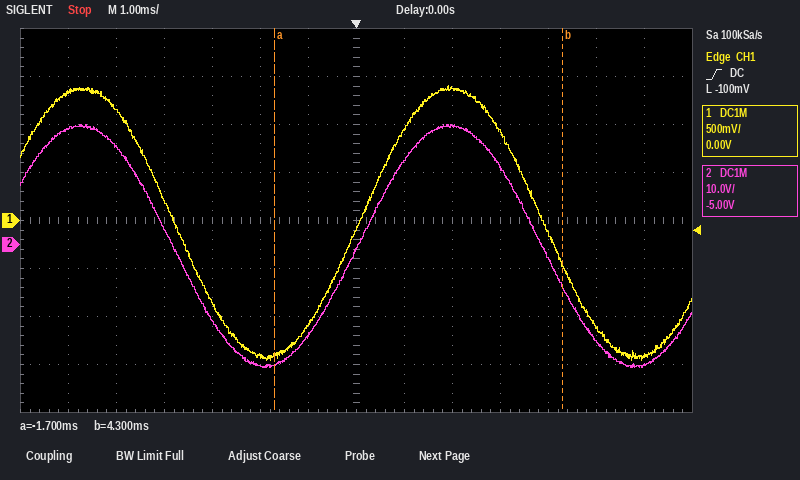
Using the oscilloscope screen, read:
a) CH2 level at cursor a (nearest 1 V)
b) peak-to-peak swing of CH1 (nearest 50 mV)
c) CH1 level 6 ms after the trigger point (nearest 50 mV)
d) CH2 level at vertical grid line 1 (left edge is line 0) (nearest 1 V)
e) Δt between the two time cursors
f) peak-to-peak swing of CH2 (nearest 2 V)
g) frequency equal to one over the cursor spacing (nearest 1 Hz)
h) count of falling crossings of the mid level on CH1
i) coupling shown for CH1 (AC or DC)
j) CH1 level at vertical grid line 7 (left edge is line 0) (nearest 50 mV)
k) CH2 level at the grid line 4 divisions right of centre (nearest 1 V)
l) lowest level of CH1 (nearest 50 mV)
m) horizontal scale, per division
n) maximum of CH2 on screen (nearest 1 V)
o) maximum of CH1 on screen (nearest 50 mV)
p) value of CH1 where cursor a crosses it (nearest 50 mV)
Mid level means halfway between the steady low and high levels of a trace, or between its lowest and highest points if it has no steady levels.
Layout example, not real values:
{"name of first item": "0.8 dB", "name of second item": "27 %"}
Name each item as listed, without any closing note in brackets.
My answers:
{"CH2 level at cursor a": "-25 V", "peak-to-peak swing of CH1": "2.85 V", "CH1 level 6 ms after the trigger point": "-1.40 V", "CH2 level at vertical grid line 1 (left edge is line 0)": "24 V", "Δt between the two time cursors": "6.0 ms", "peak-to-peak swing of CH2": "50 V", "frequency equal to one over the cursor spacing": "167 Hz", "count of falling crossings of the mid level on CH1": "2", "coupling shown for CH1": "DC", "CH1 level at vertical grid line 7 (left edge is line 0)": "-100 mV", "CH2 level at the grid line 4 divisions right of centre": "-3 V", "lowest level of CH1": "-1.45 V", "horizontal scale, per division": "1 ms", "maximum of CH2 on screen": "25 V", "maximum of CH1 on screen": "1.40 V", "value of CH1 where cursor a crosses it": "-1.40 V"}
